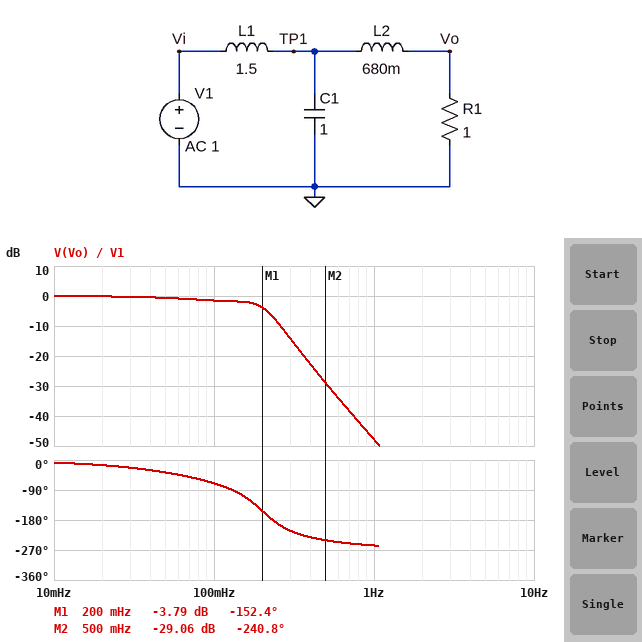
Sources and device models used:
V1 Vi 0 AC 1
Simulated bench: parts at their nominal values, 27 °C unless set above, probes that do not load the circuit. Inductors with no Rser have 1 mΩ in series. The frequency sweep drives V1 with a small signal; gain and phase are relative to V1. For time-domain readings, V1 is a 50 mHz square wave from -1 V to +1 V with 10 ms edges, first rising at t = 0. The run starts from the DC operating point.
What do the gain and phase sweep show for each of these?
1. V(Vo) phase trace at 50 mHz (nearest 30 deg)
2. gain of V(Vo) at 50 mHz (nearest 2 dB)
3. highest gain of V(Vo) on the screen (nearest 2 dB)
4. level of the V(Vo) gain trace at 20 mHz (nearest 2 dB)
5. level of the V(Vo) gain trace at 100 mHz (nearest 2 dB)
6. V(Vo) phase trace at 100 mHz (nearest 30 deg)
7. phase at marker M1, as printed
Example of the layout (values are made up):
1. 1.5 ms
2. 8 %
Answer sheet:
1. -30 deg
2. 0 dB
3. 0 dB
4. 0 dB
5. -2 dB
6. -60 deg
7. -152.4 deg
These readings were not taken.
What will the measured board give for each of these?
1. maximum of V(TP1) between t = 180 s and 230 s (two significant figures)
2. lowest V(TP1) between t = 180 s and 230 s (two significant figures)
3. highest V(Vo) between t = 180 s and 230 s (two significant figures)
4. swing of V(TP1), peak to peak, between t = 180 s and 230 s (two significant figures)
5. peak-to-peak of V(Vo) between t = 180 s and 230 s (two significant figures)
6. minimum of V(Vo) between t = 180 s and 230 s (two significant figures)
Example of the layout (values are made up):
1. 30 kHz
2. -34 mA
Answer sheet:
1. 1.1 V
2. -1.1 V
3. 1.0 V
4. 2.2 V
5. 2.0 V
6. -1.0 V
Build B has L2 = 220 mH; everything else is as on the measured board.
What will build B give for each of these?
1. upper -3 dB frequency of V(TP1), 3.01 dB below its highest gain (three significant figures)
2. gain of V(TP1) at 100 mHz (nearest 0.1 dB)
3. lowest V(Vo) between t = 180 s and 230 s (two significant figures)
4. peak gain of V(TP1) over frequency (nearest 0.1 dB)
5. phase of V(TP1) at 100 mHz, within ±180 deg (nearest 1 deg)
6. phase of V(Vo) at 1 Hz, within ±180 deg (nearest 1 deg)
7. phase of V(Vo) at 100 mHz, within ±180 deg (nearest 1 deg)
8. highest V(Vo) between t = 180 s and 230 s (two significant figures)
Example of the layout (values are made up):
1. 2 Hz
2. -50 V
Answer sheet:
1. 156 mHz
2. -0.6 dB
3. -1.1 V
4. 0 dB
5. -60 deg
6. 129 deg
7. -68 deg
8. 1.1 V
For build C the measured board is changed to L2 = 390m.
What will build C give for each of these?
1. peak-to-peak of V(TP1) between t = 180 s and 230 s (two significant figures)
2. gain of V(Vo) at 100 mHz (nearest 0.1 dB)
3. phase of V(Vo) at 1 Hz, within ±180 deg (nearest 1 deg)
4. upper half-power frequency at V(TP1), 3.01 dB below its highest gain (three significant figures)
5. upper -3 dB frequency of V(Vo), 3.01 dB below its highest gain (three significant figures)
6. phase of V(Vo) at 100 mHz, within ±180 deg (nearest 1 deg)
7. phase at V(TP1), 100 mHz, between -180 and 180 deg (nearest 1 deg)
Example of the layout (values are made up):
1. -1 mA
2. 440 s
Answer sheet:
1. 2.1 V
2. -1.0 dB
3. 114 deg
4. 176 mHz
5. 162 mHz
6. -69 deg
7. -55 deg
